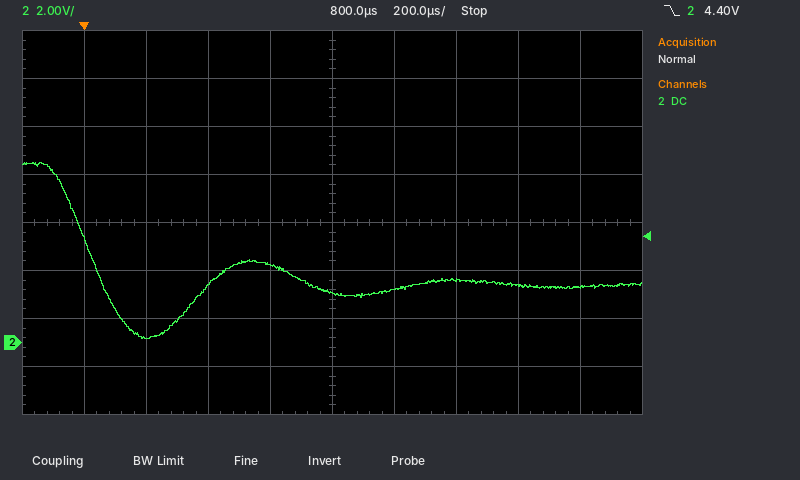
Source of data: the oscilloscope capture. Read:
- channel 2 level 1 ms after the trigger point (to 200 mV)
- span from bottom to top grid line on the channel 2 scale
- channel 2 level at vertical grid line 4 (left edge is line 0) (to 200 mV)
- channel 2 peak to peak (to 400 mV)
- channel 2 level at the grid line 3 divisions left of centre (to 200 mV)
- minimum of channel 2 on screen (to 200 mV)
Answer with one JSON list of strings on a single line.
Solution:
["2.2 V", "16 V", "3.2 V", "7.2 V", "200 mV", "200 mV"]
